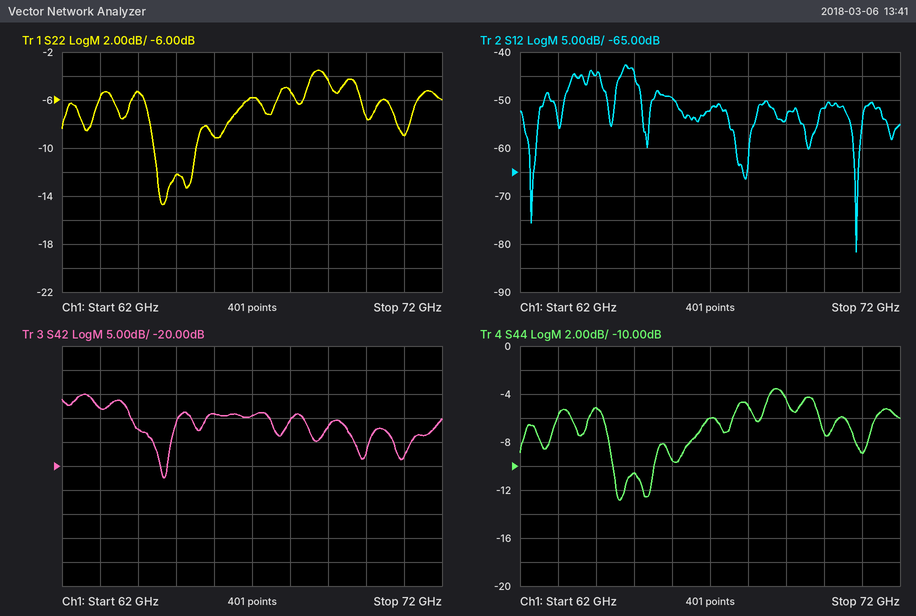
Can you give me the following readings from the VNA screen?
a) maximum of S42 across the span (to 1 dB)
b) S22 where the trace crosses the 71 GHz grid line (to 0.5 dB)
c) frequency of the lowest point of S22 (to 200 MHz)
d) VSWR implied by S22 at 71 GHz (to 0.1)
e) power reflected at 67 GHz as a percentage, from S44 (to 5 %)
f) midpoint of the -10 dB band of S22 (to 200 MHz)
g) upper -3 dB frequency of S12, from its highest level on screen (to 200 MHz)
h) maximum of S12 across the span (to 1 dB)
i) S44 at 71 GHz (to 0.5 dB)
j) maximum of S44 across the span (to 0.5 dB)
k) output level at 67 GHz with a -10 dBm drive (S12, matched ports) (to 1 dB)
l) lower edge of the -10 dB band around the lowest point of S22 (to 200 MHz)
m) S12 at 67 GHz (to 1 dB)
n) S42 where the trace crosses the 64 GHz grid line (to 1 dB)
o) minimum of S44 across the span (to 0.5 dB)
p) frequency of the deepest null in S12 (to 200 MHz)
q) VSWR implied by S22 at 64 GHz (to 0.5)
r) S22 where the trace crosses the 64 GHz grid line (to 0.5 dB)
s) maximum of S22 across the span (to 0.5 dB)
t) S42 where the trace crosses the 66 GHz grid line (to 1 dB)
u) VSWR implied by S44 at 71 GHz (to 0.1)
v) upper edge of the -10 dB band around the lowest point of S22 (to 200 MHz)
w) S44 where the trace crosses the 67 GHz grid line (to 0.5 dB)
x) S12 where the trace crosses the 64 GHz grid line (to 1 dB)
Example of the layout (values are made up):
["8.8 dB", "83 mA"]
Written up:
["-5 dB", "-9.0 dB", "64.6 GHz", "2.1", "25 %", "65.0 GHz", "65.0 GHz", "-43 dB", "-9.0 dB", "-3.5 dB", "-62 dBm", "64.4 GHz", "-52 dB", "-12 dB", "-13.0 dB", "70.8 GHz", "3.5", "-5.5 dB", "-3.5 dB", "-9 dB", "2.1", "65.6 GHz", "-6.0 dB", "-45 dB"]
